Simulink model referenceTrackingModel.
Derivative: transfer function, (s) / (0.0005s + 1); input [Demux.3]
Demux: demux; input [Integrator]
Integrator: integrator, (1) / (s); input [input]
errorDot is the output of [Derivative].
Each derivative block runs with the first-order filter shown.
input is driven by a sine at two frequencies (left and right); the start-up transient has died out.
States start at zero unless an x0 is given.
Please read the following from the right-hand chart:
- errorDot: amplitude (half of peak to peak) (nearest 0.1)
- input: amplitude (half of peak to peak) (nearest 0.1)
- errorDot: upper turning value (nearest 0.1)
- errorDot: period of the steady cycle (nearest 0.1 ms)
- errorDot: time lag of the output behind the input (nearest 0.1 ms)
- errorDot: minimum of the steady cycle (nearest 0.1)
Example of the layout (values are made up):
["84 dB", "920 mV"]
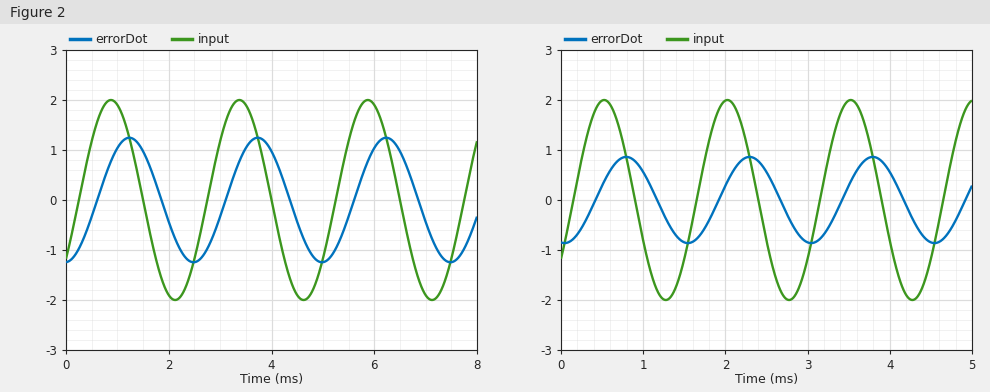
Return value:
["0.9", "2.0", "0.9", "1.5 ms", "0.3 ms", "-0.9"]
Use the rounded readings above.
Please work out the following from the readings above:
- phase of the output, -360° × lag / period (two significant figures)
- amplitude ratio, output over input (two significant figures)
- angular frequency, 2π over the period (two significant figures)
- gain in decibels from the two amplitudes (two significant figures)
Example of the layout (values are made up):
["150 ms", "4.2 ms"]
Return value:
["-72°", "0.45", "4.2 rad/ms", "-6.9 dB"]
